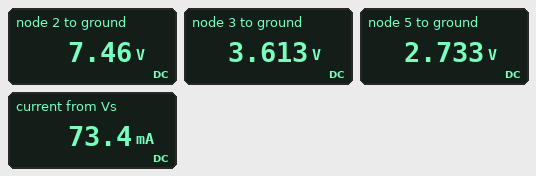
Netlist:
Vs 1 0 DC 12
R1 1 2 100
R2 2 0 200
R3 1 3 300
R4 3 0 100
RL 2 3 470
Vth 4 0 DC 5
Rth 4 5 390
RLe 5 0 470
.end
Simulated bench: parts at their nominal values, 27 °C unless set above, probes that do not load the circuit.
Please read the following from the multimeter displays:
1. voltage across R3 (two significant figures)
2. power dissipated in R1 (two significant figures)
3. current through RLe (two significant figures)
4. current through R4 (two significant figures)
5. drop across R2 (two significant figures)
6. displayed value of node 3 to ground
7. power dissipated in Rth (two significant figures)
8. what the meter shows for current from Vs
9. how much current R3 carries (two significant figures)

8.4 V
210 mW
5.8 mA
36 mA
7.5 V
3.613 V
13 mW
73.4 mA
28 mA
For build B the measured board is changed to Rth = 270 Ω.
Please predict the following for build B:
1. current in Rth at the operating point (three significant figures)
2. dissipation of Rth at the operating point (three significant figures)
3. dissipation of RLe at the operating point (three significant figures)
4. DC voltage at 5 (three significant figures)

6.76 mA
12.3 mW
21.5 mW
3.18 V
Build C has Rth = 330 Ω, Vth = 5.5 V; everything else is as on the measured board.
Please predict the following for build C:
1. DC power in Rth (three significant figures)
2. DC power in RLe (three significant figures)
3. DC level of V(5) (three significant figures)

15.6 mW
22.2 mW
3.23 V
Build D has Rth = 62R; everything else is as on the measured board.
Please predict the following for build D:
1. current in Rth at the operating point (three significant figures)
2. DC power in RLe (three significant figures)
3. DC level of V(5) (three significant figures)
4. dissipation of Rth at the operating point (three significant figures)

9.40 mA
41.5 mW
4.42 V
5.48 mW
